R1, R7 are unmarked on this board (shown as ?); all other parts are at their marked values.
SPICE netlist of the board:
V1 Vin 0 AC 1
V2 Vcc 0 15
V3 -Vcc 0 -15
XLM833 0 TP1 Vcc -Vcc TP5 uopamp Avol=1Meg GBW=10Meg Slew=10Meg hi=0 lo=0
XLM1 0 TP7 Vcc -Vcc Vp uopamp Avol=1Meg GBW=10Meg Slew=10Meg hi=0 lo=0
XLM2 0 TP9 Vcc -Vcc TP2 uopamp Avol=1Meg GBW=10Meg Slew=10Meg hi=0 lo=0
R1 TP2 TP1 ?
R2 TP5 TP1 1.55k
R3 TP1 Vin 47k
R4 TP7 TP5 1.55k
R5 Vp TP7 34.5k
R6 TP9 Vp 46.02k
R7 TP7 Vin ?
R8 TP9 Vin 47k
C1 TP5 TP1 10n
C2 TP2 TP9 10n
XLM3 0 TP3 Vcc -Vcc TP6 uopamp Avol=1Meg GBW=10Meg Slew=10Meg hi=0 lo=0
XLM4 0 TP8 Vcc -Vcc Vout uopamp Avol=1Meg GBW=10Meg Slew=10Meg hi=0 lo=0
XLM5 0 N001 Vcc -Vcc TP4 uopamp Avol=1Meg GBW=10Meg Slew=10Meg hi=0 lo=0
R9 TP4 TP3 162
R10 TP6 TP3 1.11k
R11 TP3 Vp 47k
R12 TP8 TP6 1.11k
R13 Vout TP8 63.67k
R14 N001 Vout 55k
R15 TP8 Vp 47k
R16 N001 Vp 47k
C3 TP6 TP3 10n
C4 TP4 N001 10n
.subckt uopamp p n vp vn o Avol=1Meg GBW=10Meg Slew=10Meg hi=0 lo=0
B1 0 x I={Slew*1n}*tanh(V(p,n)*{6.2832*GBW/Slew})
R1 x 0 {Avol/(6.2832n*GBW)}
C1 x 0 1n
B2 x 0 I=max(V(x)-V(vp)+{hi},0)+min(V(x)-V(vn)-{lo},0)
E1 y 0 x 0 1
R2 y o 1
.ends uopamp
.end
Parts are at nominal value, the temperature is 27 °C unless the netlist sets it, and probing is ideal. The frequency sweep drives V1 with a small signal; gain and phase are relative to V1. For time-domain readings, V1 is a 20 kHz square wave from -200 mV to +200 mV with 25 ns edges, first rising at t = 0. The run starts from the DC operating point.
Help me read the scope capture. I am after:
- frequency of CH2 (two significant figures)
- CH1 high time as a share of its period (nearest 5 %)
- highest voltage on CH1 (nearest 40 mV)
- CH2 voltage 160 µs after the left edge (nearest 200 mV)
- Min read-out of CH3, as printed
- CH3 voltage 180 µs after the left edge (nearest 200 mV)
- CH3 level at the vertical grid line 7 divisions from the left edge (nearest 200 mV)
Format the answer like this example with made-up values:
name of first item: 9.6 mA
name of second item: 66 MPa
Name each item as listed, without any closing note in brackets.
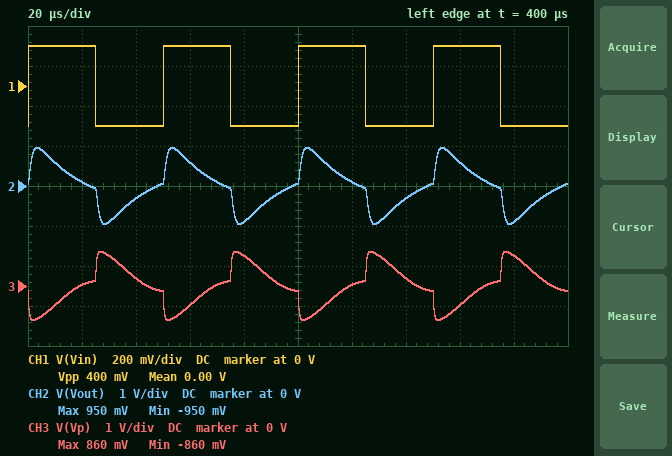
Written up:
frequency of CH2: 20 kHz
CH1 high time as a share of its period: 50 %
highest voltage on CH1: 200 mV
CH2 voltage 160 µs after the left edge: 600 mV
Min read-out of CH3, as printed: -860 mV
CH3 voltage 180 µs after the left edge: 800 mV
CH3 level at the vertical grid line 7 divisions from the left edge: 200 mV
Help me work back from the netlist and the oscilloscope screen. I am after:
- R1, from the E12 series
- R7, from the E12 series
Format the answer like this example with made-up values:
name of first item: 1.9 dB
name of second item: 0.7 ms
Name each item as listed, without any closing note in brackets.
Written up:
R1, from the E12 series: 330 Ω
R7, from the E12 series: 18 kΩ
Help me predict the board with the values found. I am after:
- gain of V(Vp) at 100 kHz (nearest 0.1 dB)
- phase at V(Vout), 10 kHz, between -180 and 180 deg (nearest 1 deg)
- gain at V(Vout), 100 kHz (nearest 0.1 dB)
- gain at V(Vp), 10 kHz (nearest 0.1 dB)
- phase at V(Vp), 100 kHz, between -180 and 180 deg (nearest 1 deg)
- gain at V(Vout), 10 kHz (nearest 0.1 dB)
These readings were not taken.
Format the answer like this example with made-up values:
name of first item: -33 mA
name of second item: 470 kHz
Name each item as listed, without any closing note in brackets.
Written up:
gain of V(Vp) at 100 kHz: 5.5 dB
phase at V(Vout), 10 kHz, between -180 and 180 deg: 10 deg
gain at V(Vout), 100 kHz: 6.6 dB
gain at V(Vp), 10 kHz: -2.7 dB
phase at V(Vp), 100 kHz, between -180 and 180 deg: 168 deg
gain at V(Vout), 10 kHz: -1.4 dB
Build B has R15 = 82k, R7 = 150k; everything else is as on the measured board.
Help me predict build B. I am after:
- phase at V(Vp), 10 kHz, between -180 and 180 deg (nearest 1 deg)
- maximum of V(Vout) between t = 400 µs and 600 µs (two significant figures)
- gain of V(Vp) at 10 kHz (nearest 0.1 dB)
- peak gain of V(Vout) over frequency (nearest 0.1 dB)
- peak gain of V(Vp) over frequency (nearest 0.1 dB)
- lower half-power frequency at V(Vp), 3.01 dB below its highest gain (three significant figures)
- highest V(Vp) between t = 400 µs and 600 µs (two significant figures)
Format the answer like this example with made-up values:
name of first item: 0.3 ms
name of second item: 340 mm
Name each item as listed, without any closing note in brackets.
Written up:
phase at V(Vp), 10 kHz, between -180 and 180 deg: 151 deg
maximum of V(Vout) between t = 400 µs and 600 µs: 520 mV
gain of V(Vp) at 10 kHz: 1.6 dB
peak gain of V(Vout) over frequency: 7.0 dB
peak gain of V(Vp) over frequency: 4.9 dB
lower half-power frequency at V(Vp), 3.01 dB below its highest gain: 10.6 kHz
highest V(Vp) between t = 400 µs and 600 µs: 390 mV
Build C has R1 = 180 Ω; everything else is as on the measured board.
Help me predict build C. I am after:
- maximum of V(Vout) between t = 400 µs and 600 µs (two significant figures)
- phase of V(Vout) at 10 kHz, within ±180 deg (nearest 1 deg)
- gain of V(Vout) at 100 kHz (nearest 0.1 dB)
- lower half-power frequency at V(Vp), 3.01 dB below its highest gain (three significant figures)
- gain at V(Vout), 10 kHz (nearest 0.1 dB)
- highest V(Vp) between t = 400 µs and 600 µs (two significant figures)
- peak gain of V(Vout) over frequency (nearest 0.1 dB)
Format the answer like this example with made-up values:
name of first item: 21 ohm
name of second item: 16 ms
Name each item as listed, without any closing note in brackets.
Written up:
maximum of V(Vout) between t = 400 µs and 600 µs: 590 mV
phase of V(Vout) at 10 kHz, within ±180 deg: -1 deg
gain of V(Vout) at 100 kHz: 6.7 dB
lower half-power frequency at V(Vp), 3.01 dB below its highest gain: 24.2 kHz
gain at V(Vout), 10 kHz: -0.3 dB
highest V(Vp) between t = 400 µs and 600 µs: 530 mV
peak gain of V(Vout) over frequency: 11.3 dB
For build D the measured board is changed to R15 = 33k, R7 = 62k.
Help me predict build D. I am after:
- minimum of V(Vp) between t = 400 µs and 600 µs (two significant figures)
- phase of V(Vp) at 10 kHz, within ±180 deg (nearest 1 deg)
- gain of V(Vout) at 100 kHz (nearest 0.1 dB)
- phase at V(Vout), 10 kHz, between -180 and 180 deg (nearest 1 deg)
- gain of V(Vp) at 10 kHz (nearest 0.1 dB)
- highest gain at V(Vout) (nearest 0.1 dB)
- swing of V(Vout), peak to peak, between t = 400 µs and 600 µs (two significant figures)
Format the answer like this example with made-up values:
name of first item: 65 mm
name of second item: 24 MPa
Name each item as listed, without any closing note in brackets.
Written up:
minimum of V(Vp) between t = 400 µs and 600 µs: -260 mV
phase of V(Vp) at 10 kHz, within ±180 deg: 156 deg
gain of V(Vout) at 100 kHz: -1.1 dB
phase at V(Vout), 10 kHz, between -180 and 180 deg: -26 deg
gain of V(Vp) at 10 kHz: 0.6 dB
highest gain at V(Vout): 7.9 dB
swing of V(Vout), peak to peak, between t = 400 µs and 600 µs: 590 mV
